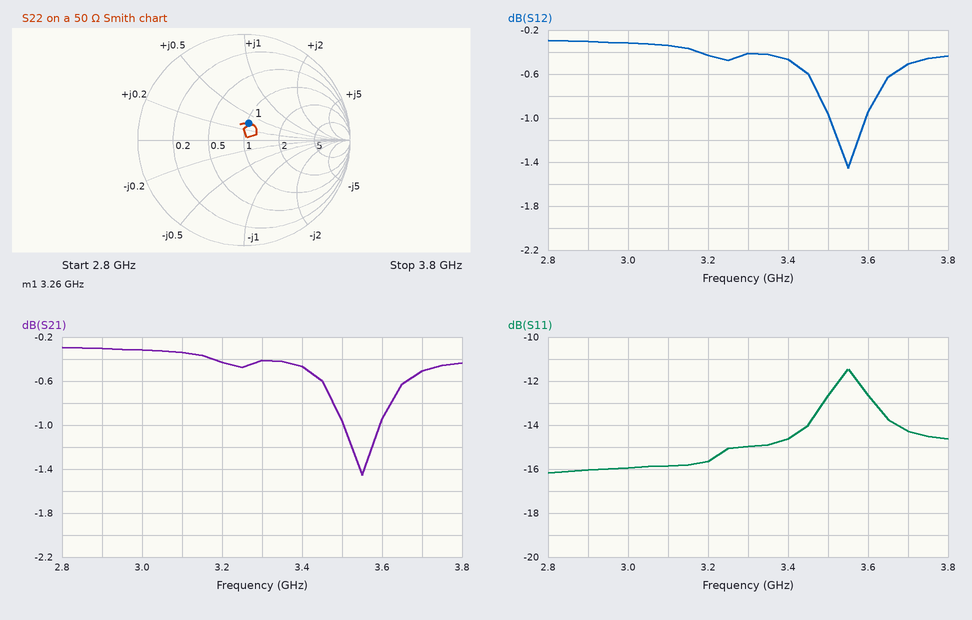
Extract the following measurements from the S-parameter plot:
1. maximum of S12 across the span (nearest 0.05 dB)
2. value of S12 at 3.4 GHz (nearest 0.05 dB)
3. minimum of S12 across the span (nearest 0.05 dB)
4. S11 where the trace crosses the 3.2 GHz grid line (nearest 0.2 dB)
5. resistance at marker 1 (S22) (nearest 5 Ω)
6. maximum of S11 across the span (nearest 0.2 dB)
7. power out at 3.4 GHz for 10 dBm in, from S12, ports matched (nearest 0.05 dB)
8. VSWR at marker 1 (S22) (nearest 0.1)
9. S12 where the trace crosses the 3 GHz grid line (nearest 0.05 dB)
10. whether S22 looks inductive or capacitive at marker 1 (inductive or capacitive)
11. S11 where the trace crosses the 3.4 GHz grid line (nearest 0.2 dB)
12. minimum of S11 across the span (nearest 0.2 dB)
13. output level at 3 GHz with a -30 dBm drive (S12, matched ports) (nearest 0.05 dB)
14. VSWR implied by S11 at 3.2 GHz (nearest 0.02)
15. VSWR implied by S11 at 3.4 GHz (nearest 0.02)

-0.30 dB
-0.45 dB
-1.45 dB
-15.6 dB
50 Ω
-11.4 dB
9.55 dBm
1.4
-0.30 dB
inductive
-14.6 dB
-16.2 dB
-30.30 dBm
1.40
1.46
